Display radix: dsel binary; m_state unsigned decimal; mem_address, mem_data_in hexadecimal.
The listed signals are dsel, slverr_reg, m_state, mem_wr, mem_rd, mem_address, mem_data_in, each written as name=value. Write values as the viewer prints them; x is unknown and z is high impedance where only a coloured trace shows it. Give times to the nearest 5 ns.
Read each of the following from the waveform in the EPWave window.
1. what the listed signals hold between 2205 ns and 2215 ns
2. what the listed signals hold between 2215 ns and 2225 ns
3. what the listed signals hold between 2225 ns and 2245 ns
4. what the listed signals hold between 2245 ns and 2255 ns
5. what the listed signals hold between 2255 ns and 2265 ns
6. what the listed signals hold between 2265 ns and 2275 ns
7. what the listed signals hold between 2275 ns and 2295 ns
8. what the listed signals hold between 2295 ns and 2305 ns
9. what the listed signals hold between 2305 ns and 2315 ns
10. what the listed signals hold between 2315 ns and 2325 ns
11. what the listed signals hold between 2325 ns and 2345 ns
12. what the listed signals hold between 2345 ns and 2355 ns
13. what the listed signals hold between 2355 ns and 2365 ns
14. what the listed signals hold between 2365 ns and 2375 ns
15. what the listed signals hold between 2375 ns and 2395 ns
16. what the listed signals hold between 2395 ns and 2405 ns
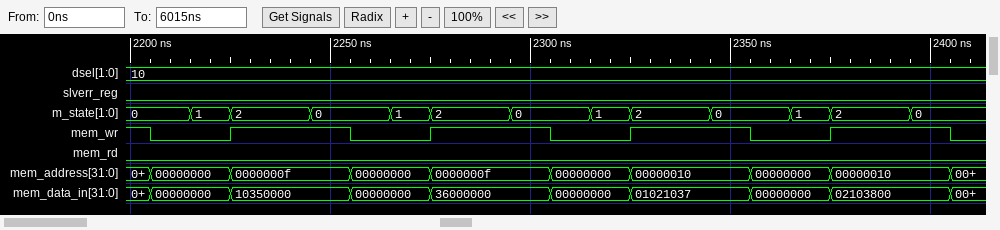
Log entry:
dsel=10, slverr_reg=0, m_state=0, mem_wr=0, mem_rd=0, mem_address=00000000, mem_data_in=00000000
dsel=10, slverr_reg=0, m_state=1, mem_wr=0, mem_rd=0, mem_address=00000000, mem_data_in=00000000
dsel=10, slverr_reg=0, m_state=2, mem_wr=1, mem_rd=0, mem_address=0000000f, mem_data_in=10350000
dsel=10, slverr_reg=0, m_state=0, mem_wr=1, mem_rd=0, mem_address=0000000f, mem_data_in=10350000
dsel=10, slverr_reg=0, m_state=0, mem_wr=0, mem_rd=0, mem_address=00000000, mem_data_in=00000000
dsel=10, slverr_reg=0, m_state=1, mem_wr=0, mem_rd=0, mem_address=00000000, mem_data_in=00000000
dsel=10, slverr_reg=0, m_state=2, mem_wr=1, mem_rd=0, mem_address=0000000f, mem_data_in=36000000
dsel=10, slverr_reg=0, m_state=0, mem_wr=1, mem_rd=0, mem_address=0000000f, mem_data_in=36000000
dsel=10, slverr_reg=0, m_state=0, mem_wr=0, mem_rd=0, mem_address=00000000, mem_data_in=00000000
dsel=10, slverr_reg=0, m_state=1, mem_wr=0, mem_rd=0, mem_address=00000000, mem_data_in=00000000
dsel=10, slverr_reg=0, m_state=2, mem_wr=1, mem_rd=0, mem_address=00000010, mem_data_in=01021037
dsel=10, slverr_reg=0, m_state=0, mem_wr=1, mem_rd=0, mem_address=00000010, mem_data_in=01021037
dsel=10, slverr_reg=0, m_state=0, mem_wr=0, mem_rd=0, mem_address=00000000, mem_data_in=00000000
dsel=10, slverr_reg=0, m_state=1, mem_wr=0, mem_rd=0, mem_address=00000000, mem_data_in=00000000
dsel=10, slverr_reg=0, m_state=2, mem_wr=1, mem_rd=0, mem_address=00000010, mem_data_in=02103800
dsel=10, slverr_reg=0, m_state=0, mem_wr=1, mem_rd=0, mem_address=00000010, mem_data_in=02103800
